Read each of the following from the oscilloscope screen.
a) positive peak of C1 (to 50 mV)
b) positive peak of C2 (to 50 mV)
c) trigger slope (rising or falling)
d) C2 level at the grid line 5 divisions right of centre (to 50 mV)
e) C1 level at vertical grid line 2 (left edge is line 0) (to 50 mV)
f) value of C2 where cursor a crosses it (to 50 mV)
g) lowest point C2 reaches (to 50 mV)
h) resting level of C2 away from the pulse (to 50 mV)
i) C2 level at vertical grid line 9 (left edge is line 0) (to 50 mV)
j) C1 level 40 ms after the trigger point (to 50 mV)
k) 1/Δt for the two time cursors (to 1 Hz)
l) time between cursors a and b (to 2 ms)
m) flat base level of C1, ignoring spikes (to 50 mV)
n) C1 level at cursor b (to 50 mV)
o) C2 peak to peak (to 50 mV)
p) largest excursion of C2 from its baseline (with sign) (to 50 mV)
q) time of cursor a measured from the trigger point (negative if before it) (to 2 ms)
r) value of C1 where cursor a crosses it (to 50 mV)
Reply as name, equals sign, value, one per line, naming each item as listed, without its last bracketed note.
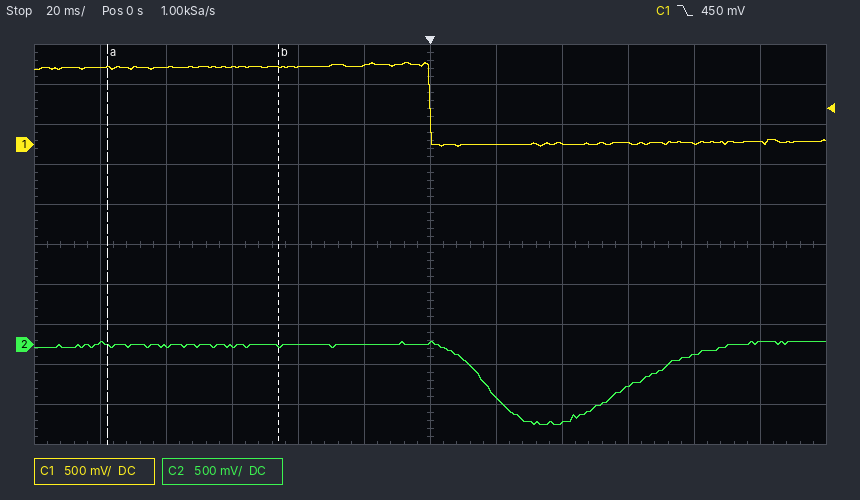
positive peak of C1 = 1.00 V
positive peak of C2 = 50 mV
trigger slope = falling
C2 level at the grid line 5 divisions right of centre = 50 mV
C1 level at vertical grid line 2 (left edge is line 0) = 950 mV
value of C2 where cursor a crosses it = 0 mV
lowest point C2 reaches = -1.00 V
resting level of C2 away from the pulse = 0 mV
C2 level at vertical grid line 9 (left edge is line 0) = -500 mV
C1 level 40 ms after the trigger point = 0 mV
1/Δt for the two time cursors = 19 Hz
time between cursors a and b = 52 ms
flat base level of C1, ignoring spikes = 0 mV
C1 level at cursor b = 950 mV
C2 peak to peak = 1.05 V
largest excursion of C2 from its baseline (with sign) = -1.00 V
time of cursor a measured from the trigger point (negative if before it) = -98 ms
value of C1 where cursor a crosses it = 950 mV
